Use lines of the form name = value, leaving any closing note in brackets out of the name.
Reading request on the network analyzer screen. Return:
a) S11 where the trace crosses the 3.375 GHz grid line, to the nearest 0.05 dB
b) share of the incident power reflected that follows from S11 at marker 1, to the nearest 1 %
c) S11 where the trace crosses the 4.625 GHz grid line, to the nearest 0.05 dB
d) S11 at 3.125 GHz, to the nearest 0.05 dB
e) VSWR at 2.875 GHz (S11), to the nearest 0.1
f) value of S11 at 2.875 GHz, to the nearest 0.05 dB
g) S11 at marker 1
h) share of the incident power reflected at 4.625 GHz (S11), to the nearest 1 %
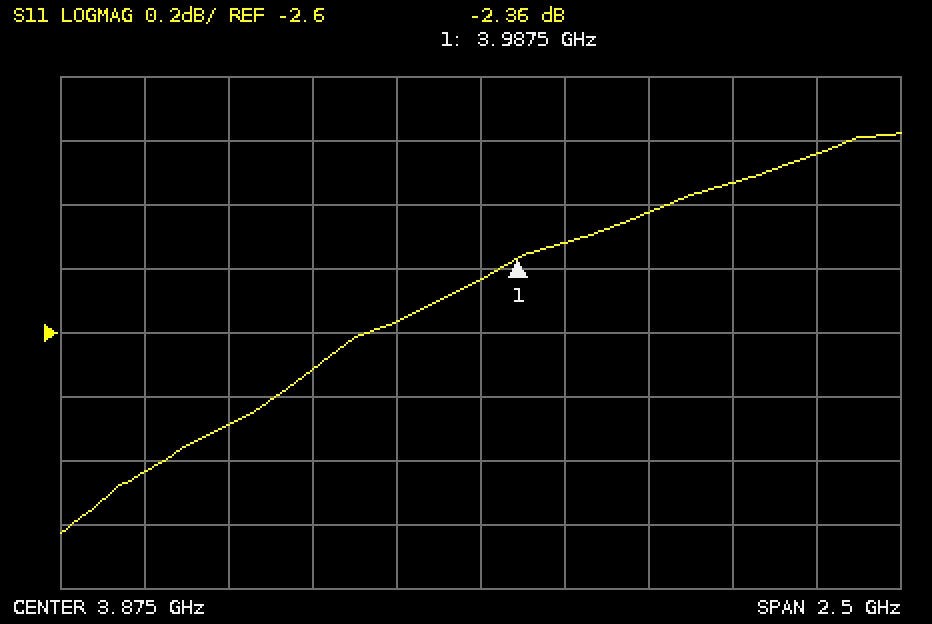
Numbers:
S11 where the trace crosses the 3.375 GHz grid line, to the nearest 0.05 dB = -2.70 dB
share of the incident power reflected that follows from S11 at marker 1, to the nearest 1 % = 58 %
S11 where the trace crosses the 4.625 GHz grid line, to the nearest 0.05 dB = -2.15 dB
S11 at 3.125 GHz, to the nearest 0.05 dB = -2.90 dB
VSWR at 2.875 GHz (S11), to the nearest 0.1 = 5.8
value of S11 at 2.875 GHz, to the nearest 0.05 dB = -3.05 dB
S11 at marker 1 = -2.36 dB
share of the incident power reflected at 4.625 GHz (S11), to the nearest 1 % = 61 %
